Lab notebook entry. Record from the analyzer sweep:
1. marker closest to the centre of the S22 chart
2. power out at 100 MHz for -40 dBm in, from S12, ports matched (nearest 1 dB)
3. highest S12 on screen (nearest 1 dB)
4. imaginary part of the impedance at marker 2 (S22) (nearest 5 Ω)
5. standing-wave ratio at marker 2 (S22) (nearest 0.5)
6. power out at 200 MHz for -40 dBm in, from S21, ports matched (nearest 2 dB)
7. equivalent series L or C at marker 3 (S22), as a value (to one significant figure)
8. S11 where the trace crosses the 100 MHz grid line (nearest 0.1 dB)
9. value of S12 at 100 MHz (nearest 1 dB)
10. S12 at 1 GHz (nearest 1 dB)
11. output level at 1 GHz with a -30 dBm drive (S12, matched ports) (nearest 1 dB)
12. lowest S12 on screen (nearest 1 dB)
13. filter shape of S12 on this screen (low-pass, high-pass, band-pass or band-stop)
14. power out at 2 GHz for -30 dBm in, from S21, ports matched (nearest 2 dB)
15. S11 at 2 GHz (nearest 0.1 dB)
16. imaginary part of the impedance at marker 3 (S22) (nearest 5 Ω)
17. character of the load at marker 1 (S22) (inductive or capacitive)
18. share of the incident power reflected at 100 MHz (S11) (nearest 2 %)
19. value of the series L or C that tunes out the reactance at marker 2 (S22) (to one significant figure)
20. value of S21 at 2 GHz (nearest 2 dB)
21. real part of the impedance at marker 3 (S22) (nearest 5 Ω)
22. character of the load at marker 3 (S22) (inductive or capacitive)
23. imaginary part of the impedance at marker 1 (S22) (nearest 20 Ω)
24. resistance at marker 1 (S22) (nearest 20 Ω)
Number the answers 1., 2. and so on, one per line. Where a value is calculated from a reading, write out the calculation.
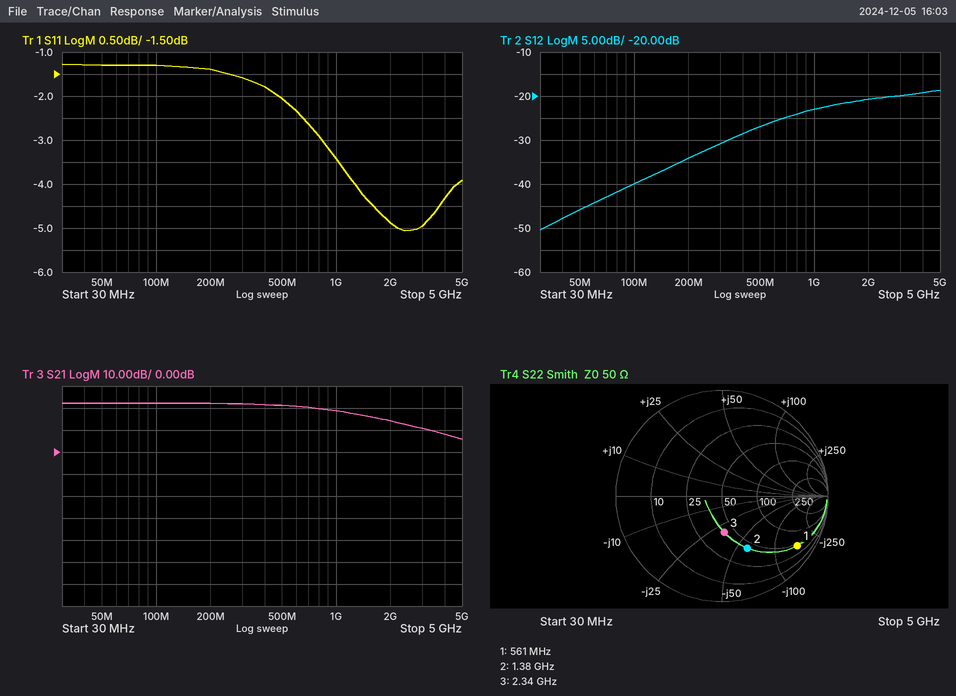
1. marker 3
2. -40 dBm + (-40 dB) = -80 dBm
3. -19 dB
4. -60 Ω
5. 3.5
6. -40 dBm + (22 dB) = -18 dBm
7. C = 1/(2π × 2.34 GHz × 30 Ω) ≈ 2 pF
8. -1.3 dB
9. -40 dB
10. -23 dB
11. -30 dBm + (-23 dB) = -53 dBm
12. -50 dB
13. high-pass
14. -30 dBm + (14 dB) = -16 dBm
15. -4.9 dB
16. -30 Ω
17. capacitive
18. 10^(-1.3/10) ≈ 74 %
19. L = 60 Ω/(2π × 1.38 GHz) ≈ 7 nH
20. 14 dB
21. 40 Ω
22. capacitive
23. -160 Ω
24. 40 Ω
